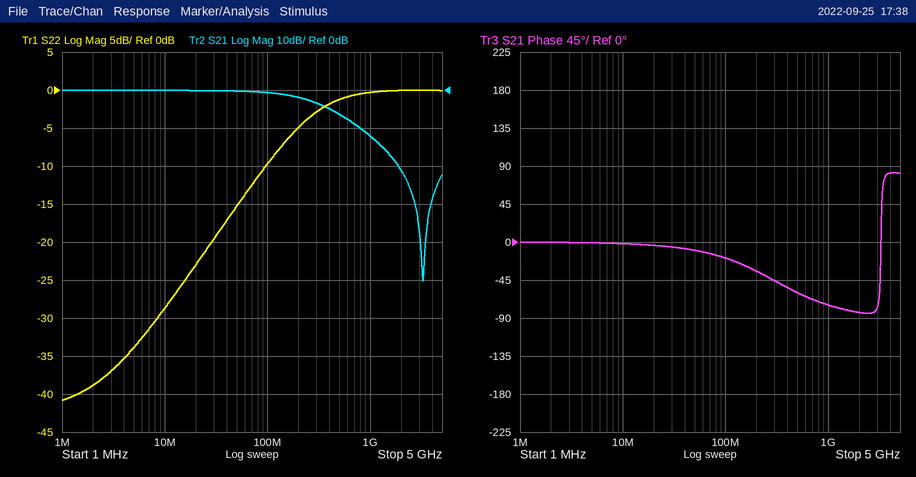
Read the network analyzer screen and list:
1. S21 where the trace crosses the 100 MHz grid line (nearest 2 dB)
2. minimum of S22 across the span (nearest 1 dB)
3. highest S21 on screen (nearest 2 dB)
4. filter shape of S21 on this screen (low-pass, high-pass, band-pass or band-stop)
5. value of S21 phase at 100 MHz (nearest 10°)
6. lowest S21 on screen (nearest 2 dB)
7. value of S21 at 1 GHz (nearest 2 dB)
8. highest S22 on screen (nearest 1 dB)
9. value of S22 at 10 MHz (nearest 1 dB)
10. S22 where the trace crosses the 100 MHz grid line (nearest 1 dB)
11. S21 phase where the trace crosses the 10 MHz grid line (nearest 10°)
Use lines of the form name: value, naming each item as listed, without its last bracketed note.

S21 where the trace crosses the 100 MHz grid line: 0 dB
minimum of S22 across the span: -41 dB
highest S21 on screen: 0 dB
filter shape of S21 on this screen: low-pass
value of S21 phase at 100 MHz: -20°
lowest S21 on screen: -50 dB
value of S21 at 1 GHz: -12 dB
highest S22 on screen: 0 dB
value of S22 at 10 MHz: -29 dB
S22 where the trace crosses the 100 MHz grid line: -10 dB
S21 phase where the trace crosses the 10 MHz grid line: 0°
